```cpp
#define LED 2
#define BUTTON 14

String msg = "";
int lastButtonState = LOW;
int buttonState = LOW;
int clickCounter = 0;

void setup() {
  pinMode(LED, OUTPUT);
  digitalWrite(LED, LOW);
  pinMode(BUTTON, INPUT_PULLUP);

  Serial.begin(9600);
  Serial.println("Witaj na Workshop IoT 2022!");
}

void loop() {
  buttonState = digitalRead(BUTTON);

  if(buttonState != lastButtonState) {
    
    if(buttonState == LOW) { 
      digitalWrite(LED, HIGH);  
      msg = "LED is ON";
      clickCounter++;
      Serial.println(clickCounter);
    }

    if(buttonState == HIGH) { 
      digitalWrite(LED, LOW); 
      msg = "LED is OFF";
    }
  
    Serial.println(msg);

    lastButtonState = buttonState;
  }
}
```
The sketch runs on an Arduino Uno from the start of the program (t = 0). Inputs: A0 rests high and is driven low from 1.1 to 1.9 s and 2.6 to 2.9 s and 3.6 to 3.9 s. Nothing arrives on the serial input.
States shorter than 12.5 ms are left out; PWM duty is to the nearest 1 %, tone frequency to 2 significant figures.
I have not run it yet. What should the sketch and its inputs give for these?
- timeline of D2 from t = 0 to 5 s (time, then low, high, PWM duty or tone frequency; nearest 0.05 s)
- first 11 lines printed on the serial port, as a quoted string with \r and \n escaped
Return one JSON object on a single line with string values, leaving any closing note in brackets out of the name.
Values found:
{"timeline of D2 from t = 0 to 5 s": "0 s low; 1.1 s high; 1.9 s low; 2.6 s high; 2.9 s low; 3.6 s high; 3.9 s low", "first 11 lines printed on the serial port, as a quoted string with \\r and \\n escaped": "\"Witaj na Workshop IoT 2022!\\r\\nLED is OFF\\r\\n1\\r\\nLED is ON\\r\\nLED is OFF\\r\\n2\\r\\nLED is ON\\r\\nLED is OFF\\r\\n3\\r\\nLED is ON\\r\\nLED is OFF\\r\\n\""}
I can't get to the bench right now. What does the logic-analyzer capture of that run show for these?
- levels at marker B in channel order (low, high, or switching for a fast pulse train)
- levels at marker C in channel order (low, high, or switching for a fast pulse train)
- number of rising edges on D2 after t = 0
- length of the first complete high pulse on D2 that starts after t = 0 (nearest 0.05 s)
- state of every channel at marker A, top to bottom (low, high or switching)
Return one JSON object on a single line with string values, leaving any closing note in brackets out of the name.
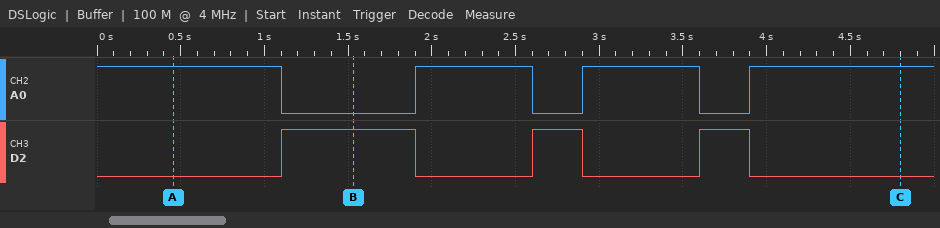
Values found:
{"levels at marker B in channel order": "A0 low, D2 high", "levels at marker C in channel order": "A0 high, D2 low", "number of rising edges on D2 after t = 0": "3", "length of the first complete high pulse on D2 that starts after t = 0": "0.80 s", "state of every channel at marker A, top to bottom": "A0 high, D2 low"}
